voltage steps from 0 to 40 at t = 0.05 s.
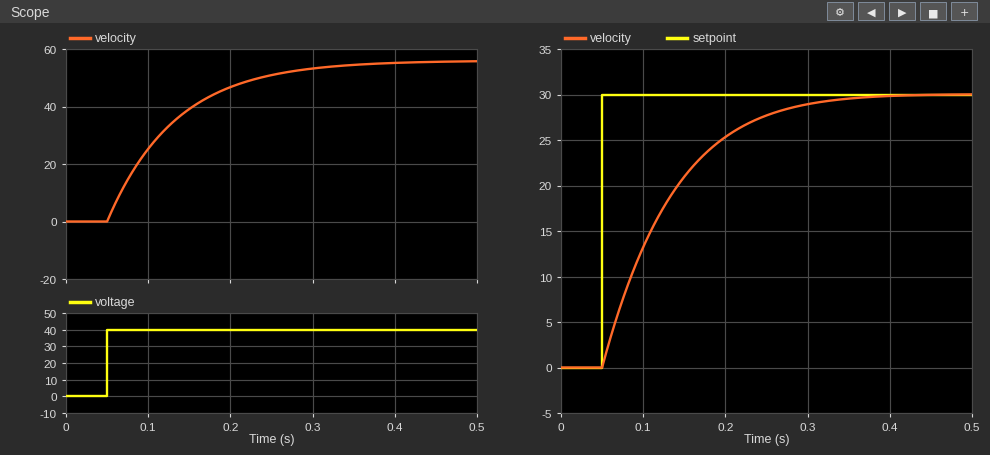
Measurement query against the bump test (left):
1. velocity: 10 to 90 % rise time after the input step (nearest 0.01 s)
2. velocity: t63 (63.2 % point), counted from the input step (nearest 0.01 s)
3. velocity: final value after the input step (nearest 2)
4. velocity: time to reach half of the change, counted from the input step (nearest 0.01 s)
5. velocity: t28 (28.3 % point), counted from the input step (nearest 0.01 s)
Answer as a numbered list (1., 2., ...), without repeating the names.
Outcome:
1. 0.18 s
2. 0.08 s
3. 56
4. 0.06 s
5. 0.03 s
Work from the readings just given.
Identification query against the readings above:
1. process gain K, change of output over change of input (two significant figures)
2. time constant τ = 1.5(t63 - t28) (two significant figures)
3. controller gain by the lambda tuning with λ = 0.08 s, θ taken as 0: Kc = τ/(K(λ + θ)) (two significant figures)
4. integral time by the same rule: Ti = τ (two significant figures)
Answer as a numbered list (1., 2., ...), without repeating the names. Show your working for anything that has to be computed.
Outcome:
1. (56 - 0) / 40 = 1.4
2. 1.5 × (0.08 - 0.03) = 0.075 s
3. 0.075 / (1.4 × (0.08 + 0)) = 0.67
4. 0.075 s
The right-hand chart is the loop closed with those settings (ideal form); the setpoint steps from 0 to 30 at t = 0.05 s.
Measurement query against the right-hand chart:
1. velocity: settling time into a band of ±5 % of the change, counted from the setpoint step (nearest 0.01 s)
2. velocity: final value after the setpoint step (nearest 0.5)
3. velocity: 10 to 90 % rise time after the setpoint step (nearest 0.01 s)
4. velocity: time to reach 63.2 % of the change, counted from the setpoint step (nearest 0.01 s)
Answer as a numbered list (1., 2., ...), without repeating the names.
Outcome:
1. 0.23 s
2. 30.0
3. 0.17 s
4. 0.08 s
